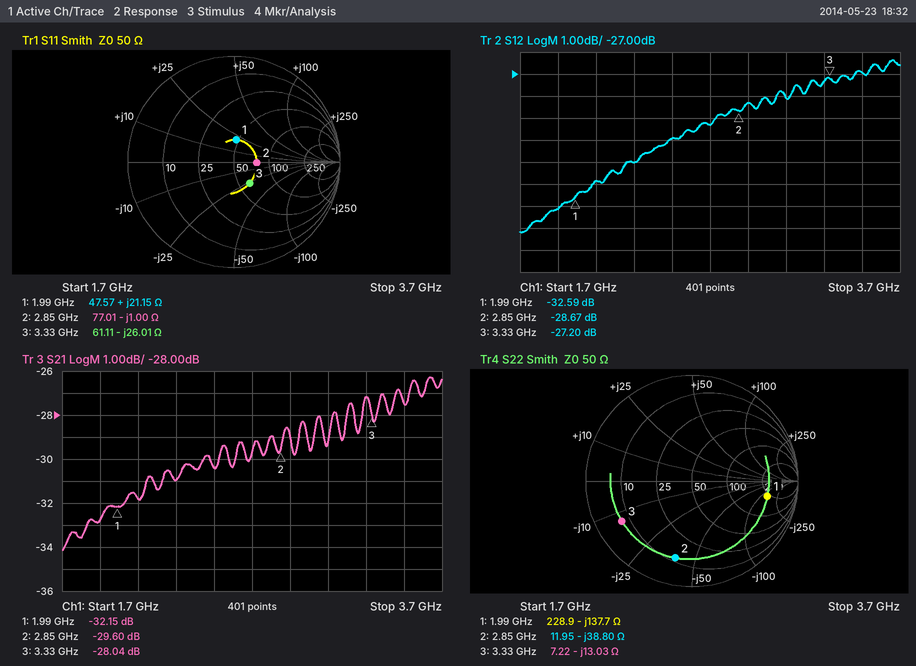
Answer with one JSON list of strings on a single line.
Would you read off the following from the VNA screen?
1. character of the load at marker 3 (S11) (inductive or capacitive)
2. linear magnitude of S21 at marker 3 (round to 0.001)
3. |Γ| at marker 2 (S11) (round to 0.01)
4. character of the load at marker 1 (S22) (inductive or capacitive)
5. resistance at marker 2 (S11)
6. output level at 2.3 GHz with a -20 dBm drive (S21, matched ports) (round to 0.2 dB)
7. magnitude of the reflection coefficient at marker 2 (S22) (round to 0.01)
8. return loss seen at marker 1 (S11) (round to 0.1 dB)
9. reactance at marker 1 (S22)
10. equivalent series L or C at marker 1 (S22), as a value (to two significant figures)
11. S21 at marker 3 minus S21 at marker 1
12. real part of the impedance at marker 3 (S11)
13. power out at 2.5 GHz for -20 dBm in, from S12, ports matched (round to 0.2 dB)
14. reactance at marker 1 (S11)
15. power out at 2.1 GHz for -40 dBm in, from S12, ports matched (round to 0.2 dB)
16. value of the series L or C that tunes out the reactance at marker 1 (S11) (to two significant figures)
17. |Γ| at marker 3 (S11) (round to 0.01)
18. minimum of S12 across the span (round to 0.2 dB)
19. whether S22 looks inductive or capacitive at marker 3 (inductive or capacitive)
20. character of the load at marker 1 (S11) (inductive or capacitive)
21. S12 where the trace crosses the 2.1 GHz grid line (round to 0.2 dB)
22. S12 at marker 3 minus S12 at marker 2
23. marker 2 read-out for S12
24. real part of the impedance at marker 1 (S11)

["capacitive", "0.040", "0.21", "capacitive", "77.01 Ω", "-51.0 dBm", "0.74", "13.4 dB", "-137.7 Ω", "580 fF", "4.11 dB", "61.11 Ω", "-50.0 dBm", "+21.15 Ω", "-71.8 dBm", "3.8 pF", "0.25", "-34.2 dB", "capacitive", "inductive", "-31.8 dB", "1.47 dB", "-28.67 dB", "47.57 Ω"]
